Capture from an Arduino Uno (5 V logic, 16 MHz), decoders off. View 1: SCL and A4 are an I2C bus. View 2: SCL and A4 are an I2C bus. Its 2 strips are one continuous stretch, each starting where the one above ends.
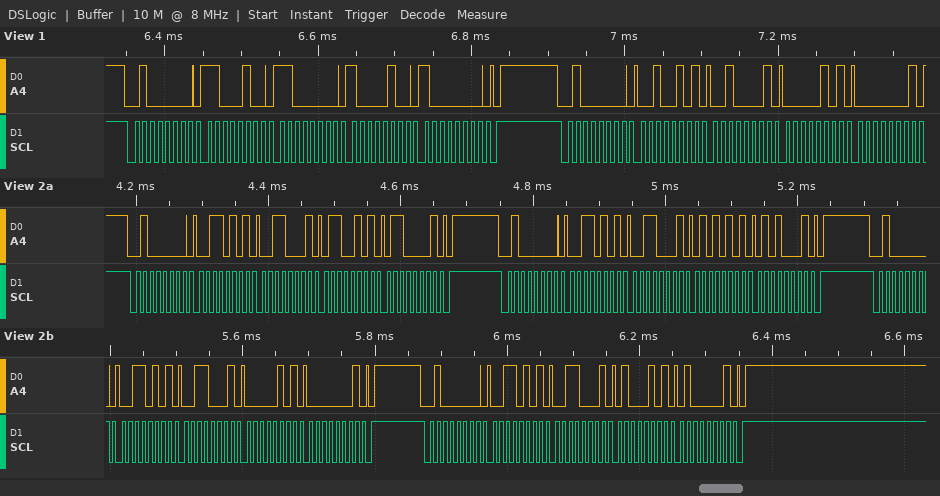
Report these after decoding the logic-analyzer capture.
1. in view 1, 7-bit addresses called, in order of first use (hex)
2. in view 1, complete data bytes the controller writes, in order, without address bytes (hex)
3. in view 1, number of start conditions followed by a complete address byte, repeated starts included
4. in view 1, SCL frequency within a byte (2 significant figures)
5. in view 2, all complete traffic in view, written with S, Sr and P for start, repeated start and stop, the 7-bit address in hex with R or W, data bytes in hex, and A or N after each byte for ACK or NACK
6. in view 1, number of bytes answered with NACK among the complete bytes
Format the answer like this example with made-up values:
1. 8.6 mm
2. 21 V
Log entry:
1. 0x20
2. C4 C0 84 80 25 21 05 01
3. 2
4. 100 kHz
5. S 20W A 35 A 31 A 65 A 61 A P S 20W A 35 A 31 A 55 A 51 A P S 20W A 35 A 31 A 05 A 01 A P S 20W A 35 A 31 A 45 A 41 A P
6. 0
